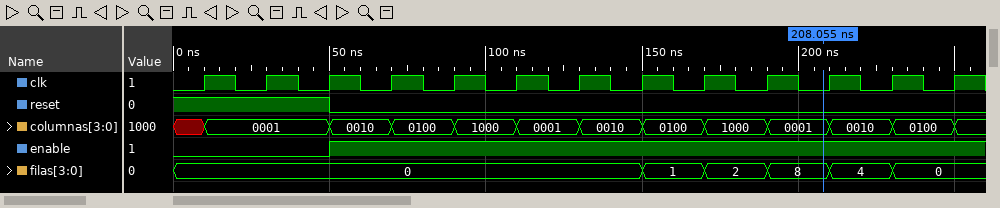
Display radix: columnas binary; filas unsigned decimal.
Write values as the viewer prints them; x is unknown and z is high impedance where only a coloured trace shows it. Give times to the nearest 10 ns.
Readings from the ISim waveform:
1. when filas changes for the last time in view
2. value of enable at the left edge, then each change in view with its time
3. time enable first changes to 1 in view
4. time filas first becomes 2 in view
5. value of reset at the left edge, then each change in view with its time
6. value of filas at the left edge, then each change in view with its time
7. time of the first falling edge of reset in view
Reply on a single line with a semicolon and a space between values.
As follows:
230 ns; 0, 1 at 50 ns; 50 ns; 170 ns; 1, 0 at 50 ns; 0, 1 at 150 ns, 2 at 170 ns, 8 at 190 ns, 4 at 210 ns, 0 at 230 ns; 50 ns
